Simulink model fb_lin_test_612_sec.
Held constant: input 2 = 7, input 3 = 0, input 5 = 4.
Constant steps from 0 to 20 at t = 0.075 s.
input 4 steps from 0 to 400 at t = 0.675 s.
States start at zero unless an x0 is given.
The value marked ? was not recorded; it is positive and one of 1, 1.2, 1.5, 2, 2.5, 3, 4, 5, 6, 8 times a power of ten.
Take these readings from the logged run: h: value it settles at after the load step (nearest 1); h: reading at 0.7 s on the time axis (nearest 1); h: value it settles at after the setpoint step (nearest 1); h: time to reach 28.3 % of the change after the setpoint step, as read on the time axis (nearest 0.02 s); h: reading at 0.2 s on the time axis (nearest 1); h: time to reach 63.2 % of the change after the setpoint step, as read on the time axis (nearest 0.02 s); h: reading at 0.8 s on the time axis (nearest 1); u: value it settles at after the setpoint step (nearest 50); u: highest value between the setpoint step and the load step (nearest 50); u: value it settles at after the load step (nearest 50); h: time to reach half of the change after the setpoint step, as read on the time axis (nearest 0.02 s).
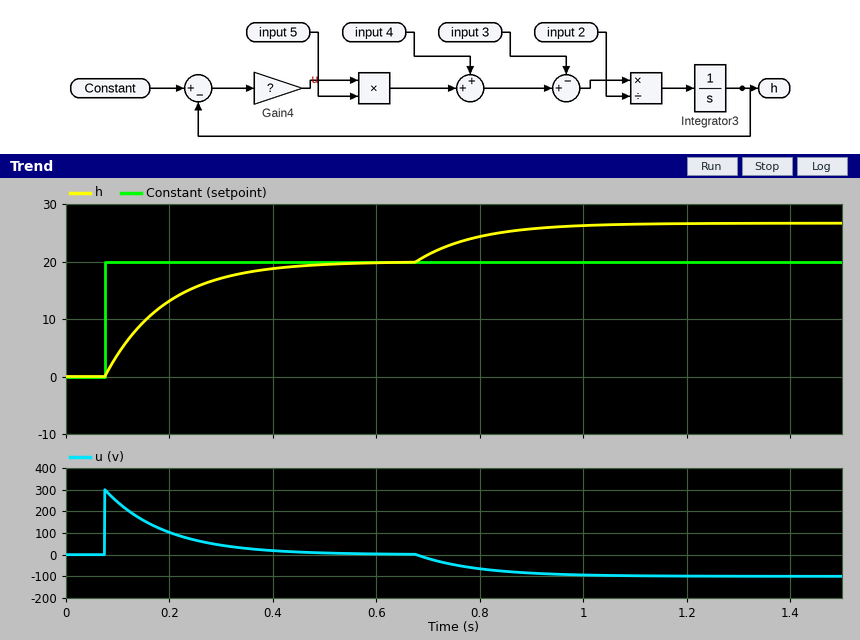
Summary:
27
21
20
0.12 s
13
0.20 s
24
0
300
-100
0.16 s
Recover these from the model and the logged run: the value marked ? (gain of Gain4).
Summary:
15
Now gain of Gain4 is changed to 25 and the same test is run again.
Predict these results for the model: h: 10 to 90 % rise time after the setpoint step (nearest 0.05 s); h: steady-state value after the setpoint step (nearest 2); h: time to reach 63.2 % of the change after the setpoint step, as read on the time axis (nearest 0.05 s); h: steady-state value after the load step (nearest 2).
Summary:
0.15 s
20
0.15 s
24
